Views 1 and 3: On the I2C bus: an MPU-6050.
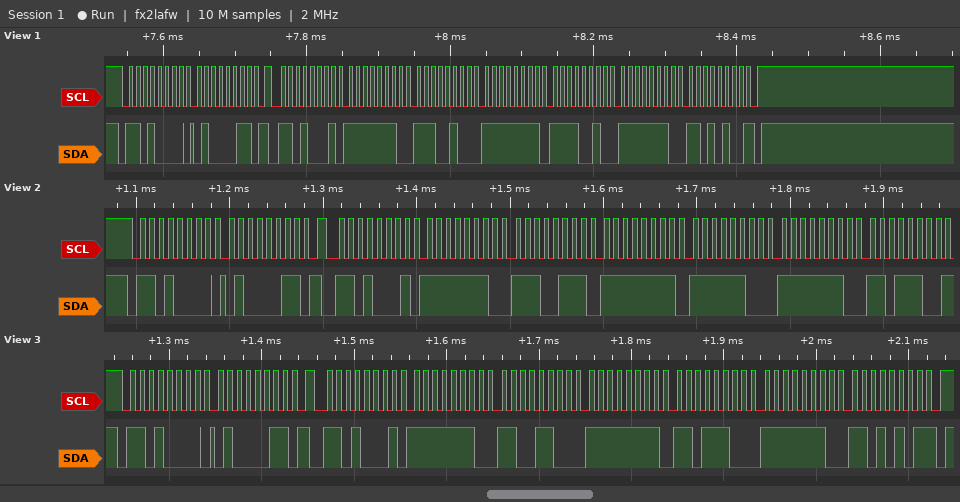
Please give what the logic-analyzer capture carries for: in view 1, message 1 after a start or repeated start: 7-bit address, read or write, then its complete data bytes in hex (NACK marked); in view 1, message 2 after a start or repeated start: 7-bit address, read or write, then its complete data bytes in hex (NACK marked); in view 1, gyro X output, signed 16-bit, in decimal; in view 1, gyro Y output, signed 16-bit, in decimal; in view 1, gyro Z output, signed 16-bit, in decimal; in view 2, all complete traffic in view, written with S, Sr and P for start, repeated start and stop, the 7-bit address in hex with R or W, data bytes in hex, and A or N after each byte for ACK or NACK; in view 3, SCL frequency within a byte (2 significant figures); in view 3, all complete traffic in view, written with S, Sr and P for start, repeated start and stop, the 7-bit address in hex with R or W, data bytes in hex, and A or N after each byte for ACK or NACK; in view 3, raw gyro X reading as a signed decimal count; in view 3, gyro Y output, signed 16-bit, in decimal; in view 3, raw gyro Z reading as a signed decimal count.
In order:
0x68 write: 43
0x68 read: FE E4 FF F2 FE D4 NACK
-284
-14
-300
S 68W A 43 A Sr 68R A FE A E7 A FF A FC A FE A DC N
100 kHz
S 68W A 43 A Sr 68R A FE A CC A FF A DC A FE A D5 N P
-308
-36
-299
